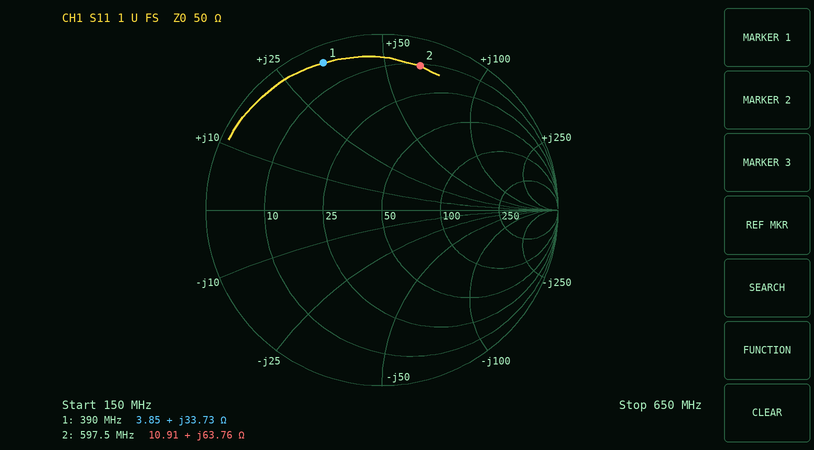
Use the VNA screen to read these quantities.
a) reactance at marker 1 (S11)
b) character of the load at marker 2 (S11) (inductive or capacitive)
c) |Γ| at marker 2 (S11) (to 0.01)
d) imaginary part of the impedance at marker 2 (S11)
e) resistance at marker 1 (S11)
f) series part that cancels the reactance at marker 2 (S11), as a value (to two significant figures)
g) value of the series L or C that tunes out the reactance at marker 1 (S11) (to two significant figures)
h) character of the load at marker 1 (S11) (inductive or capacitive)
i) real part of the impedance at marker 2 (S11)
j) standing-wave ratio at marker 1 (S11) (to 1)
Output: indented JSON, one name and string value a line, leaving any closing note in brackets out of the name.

{
  "reactance at marker 1": "+33.73 Ω",
  "character of the load at marker 2 (S11)": "inductive",
  "|Γ| at marker 2 (S11)": "0.85",
  "imaginary part of the impedance at marker 2": "+63.76 Ω",
  "resistance at marker 1": "3.85 Ω",
  "series part that cancels the reactance at marker 2 (S11), as a value": "4.2 pF",
  "value of the series L or C that tunes out the reactance at marker 1 (S11)": "12 pF",
  "character of the load at marker 1 (S11)": "inductive",
  "real part of the impedance at marker 2": "10.91 Ω",
  "standing-wave ratio at marker 1 (S11)": "19"
}
